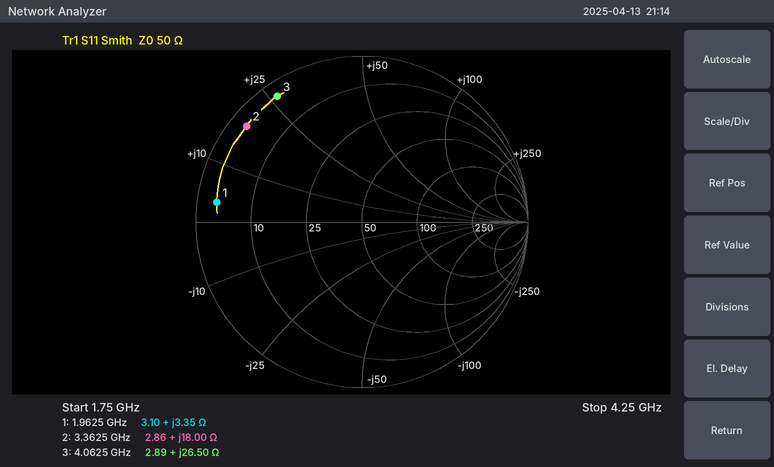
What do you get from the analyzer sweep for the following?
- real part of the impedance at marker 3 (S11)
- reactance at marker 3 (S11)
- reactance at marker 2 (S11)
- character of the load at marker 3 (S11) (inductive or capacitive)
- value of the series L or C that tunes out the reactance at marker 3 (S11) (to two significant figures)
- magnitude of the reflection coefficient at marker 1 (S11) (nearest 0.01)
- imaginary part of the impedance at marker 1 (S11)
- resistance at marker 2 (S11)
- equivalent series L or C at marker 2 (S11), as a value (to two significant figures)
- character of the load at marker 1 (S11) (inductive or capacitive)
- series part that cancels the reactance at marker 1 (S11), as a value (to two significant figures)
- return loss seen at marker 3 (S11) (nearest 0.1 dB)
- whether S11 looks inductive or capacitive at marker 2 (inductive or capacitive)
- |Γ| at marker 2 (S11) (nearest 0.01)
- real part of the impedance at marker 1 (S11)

2.89 Ω
+26.50 Ω
+18.00 Ω
inductive
1.5 pF
0.88
+3.35 Ω
2.86 Ω
850 pH
inductive
24 pF
0.8 dB
inductive
0.90
3.10 Ω
